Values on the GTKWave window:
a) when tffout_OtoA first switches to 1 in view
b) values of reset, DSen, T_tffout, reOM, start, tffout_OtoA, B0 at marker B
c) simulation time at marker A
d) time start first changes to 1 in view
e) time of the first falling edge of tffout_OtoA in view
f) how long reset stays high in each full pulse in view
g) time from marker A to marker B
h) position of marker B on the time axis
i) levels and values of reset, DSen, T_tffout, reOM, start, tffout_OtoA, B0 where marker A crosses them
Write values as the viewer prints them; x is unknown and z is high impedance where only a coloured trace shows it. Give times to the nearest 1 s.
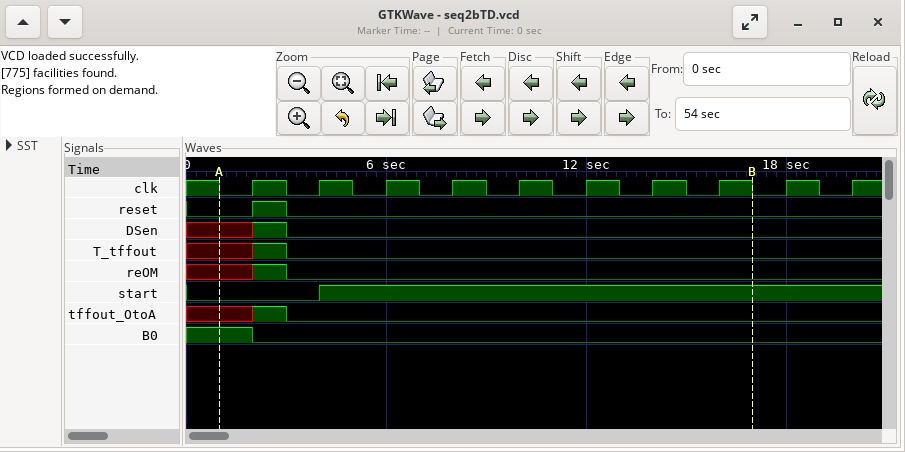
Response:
2 s
reset=0, DSen=0, T_tffout=0, reOM=0, start=1, tffout_OtoA=0, B0=0
1 s
4 s
3 s
1 s
16 s
17 s
reset=0, DSen=x, T_tffout=x, reOM=x, start=0, tffout_OtoA=x, B0=1
